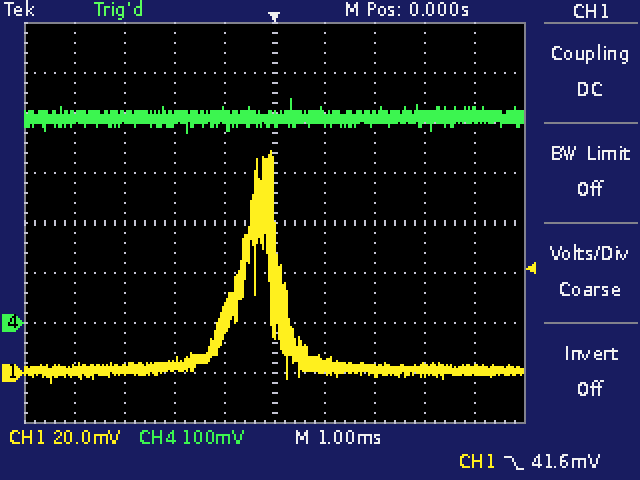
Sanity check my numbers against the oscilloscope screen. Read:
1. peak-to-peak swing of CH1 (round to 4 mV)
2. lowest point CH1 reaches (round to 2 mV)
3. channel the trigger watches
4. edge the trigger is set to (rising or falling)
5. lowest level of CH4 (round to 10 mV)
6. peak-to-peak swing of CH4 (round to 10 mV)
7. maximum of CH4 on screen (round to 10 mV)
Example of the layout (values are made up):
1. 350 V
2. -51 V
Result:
1. 92 mV
2. -4 mV
3. CH1
4. falling
5. 380 mV
6. 70 mV
7. 450 mV
